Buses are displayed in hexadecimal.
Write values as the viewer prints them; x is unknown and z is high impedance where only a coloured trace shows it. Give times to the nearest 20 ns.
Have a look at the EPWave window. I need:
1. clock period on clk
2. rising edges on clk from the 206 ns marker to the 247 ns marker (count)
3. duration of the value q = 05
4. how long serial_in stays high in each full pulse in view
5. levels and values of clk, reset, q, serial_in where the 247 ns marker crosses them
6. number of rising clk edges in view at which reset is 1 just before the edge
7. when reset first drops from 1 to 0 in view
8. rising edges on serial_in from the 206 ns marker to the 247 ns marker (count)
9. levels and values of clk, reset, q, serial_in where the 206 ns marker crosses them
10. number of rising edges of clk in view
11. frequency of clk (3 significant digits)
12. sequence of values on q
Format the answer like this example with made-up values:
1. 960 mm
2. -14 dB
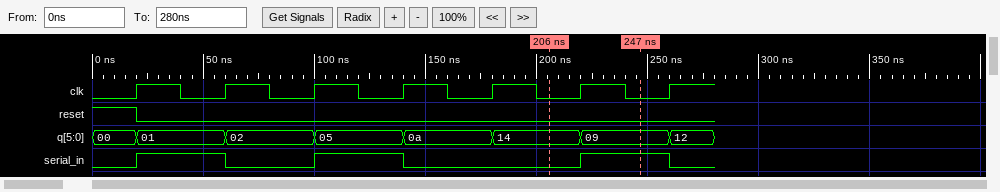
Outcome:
1. 40 ns
2. 1
3. 40 ns
4. 40 ns, 40 ns, 40 ns
5. clk=0, reset=0, q=09, serial_in=1
6. 1
7. 20 ns
8. 1
9. clk=0, reset=0, q=14, serial_in=0
10. 7
11. 25.0 MHz
12. 00, 01, 02, 05, 0a, 14, 09, 12
